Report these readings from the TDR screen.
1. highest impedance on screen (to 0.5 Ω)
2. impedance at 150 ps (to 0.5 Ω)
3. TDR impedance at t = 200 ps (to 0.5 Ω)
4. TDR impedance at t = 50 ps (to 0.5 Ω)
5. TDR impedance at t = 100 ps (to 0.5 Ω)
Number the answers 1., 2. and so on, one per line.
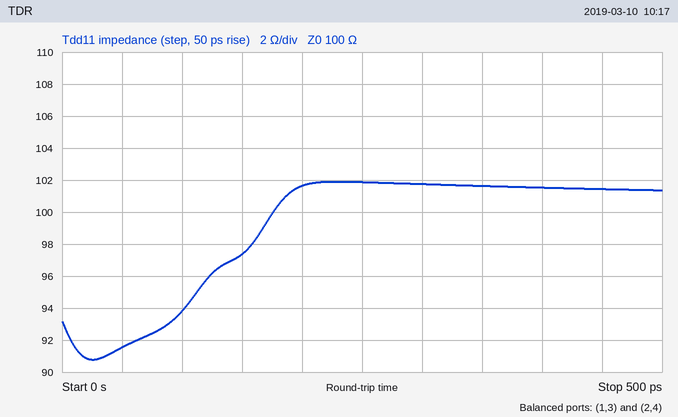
1. 102.0 Ω
2. 97.5 Ω
3. 101.5 Ω
4. 91.5 Ω
5. 94.0 Ω
